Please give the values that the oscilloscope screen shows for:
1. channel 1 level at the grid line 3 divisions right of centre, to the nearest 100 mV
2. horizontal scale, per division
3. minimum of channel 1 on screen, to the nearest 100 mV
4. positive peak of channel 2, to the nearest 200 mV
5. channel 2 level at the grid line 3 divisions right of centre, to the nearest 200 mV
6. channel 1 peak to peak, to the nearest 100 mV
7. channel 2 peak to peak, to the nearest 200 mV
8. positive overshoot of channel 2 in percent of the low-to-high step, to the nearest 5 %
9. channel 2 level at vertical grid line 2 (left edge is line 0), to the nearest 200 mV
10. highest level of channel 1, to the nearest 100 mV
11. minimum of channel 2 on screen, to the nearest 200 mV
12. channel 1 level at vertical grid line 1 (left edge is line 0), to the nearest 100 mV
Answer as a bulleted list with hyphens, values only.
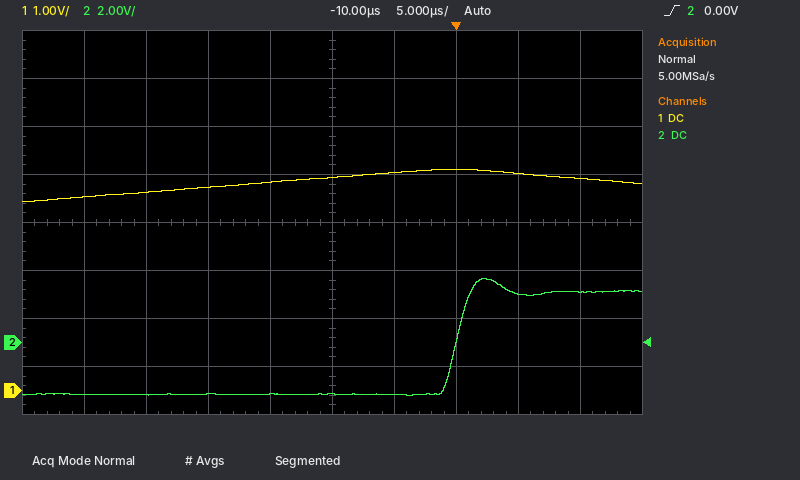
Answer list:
- 4.5 V
- 5 µs
- 3.9 V
- 2.6 V
- 2.0 V
- 700 mV
- 4.8 V
- 15 %
- -2.2 V
- 4.6 V
- -2.2 V
- 4.0 V
